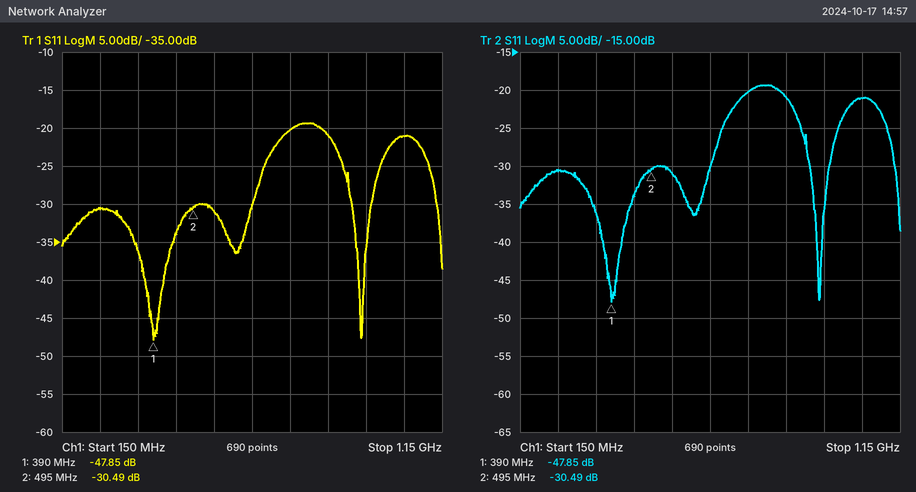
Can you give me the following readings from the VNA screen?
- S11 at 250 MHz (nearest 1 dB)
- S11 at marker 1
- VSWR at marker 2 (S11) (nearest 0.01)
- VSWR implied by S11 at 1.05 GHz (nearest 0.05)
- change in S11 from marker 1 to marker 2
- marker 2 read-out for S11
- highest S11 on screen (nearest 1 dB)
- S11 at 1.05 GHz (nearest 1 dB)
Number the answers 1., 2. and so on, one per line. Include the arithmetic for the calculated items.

1. -31 dB
2. -47.85 dB
3. (1 + 0.0299)/(1 − 0.0299) ≈ 1.06
4. |Γ| = 10^(-21/20) = 0.0891; VSWR = (1 + 0.0891)/(1 − 0.0891) ≈ 1.20
5. -30.49 − (-47.85) = 17.36 dB
6. -30.49 dB
7. -19 dB
8. -21 dB
